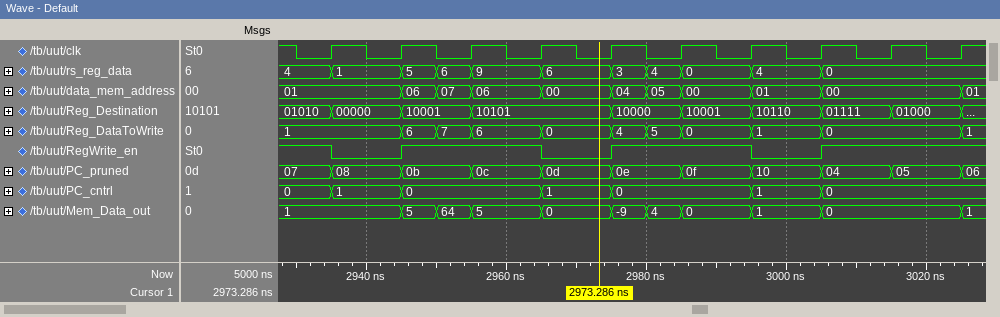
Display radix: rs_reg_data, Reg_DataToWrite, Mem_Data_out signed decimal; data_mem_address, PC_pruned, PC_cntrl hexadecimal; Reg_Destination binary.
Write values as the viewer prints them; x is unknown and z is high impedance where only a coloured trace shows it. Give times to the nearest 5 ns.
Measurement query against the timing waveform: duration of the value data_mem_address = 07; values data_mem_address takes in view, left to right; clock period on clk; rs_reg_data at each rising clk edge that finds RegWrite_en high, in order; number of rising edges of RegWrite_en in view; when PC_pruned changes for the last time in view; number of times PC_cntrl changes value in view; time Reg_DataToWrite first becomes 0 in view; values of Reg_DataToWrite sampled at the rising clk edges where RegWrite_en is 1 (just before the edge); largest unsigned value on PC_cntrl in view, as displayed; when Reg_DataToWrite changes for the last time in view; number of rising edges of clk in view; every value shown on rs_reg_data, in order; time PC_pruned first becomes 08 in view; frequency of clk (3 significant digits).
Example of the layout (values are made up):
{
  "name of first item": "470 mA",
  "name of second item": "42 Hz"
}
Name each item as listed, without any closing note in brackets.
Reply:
{
  "duration of the value data_mem_address = 07": "5 ns",
  "values data_mem_address takes in view, left to right": "01, 06, 07, 06, 00, 04, 05, 00, 01, 00, 01",
  "clock period on clk": "10 ns",
  "rs_reg_data at each rising clk edge that finds RegWrite_en high, in order": "4, 6, 9, 4, 0, 0, 0",
  "number of rising edges of RegWrite_en in view": "3",
  "when PC_pruned changes for the last time in view": "3025 ns",
  "number of times PC_cntrl changes value in view": "6",
  "time Reg_DataToWrite first becomes 0 in view": "2965 ns",
  "values of Reg_DataToWrite sampled at the rising clk edges where RegWrite_en is 1": "1, 7, 6, 5, 0, 0, 0",
  "largest unsigned value on PC_cntrl in view, as displayed": "1",
  "when Reg_DataToWrite changes for the last time in view": "3025 ns",
  "number of rising edges of clk in view": "10",
  "every value shown on rs_reg_data, in order": "4, 1, 5, 6, 9, 6, 3, 4, 0, 4, 0",
  "time PC_pruned first becomes 08 in view": "2935 ns",
  "frequency of clk": "100 MHz"
}
